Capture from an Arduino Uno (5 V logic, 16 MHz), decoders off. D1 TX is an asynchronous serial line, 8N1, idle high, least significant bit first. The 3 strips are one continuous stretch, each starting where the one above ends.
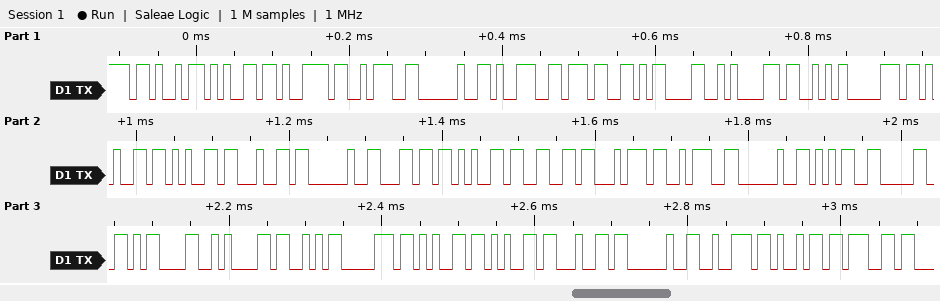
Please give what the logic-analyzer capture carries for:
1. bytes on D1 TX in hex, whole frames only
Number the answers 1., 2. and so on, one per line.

1. 4B 65 79 3A 20 39 37 0D 0A 53 70 65 65 64 20 6C 65 66 74 3A 20 35 30 0D 0A 53 70 65 65 64 20 72 69 67
